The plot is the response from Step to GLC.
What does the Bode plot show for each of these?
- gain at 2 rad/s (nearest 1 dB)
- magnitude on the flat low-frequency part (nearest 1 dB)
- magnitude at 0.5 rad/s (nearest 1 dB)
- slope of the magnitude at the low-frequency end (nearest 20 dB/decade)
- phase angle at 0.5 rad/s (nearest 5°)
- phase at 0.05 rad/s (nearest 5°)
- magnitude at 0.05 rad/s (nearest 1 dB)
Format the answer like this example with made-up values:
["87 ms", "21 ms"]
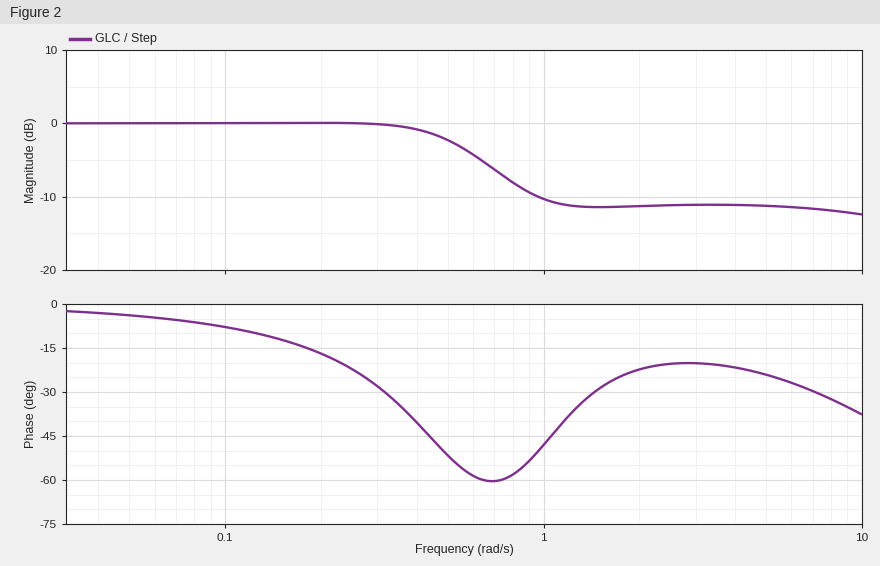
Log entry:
["-11 dB", "0 dB", "-2 dB", "0 dB/decade", "-50°", "-5°", "0 dB"]
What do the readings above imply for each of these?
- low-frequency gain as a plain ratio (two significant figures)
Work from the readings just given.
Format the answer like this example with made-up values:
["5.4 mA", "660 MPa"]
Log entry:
["1.0"]
